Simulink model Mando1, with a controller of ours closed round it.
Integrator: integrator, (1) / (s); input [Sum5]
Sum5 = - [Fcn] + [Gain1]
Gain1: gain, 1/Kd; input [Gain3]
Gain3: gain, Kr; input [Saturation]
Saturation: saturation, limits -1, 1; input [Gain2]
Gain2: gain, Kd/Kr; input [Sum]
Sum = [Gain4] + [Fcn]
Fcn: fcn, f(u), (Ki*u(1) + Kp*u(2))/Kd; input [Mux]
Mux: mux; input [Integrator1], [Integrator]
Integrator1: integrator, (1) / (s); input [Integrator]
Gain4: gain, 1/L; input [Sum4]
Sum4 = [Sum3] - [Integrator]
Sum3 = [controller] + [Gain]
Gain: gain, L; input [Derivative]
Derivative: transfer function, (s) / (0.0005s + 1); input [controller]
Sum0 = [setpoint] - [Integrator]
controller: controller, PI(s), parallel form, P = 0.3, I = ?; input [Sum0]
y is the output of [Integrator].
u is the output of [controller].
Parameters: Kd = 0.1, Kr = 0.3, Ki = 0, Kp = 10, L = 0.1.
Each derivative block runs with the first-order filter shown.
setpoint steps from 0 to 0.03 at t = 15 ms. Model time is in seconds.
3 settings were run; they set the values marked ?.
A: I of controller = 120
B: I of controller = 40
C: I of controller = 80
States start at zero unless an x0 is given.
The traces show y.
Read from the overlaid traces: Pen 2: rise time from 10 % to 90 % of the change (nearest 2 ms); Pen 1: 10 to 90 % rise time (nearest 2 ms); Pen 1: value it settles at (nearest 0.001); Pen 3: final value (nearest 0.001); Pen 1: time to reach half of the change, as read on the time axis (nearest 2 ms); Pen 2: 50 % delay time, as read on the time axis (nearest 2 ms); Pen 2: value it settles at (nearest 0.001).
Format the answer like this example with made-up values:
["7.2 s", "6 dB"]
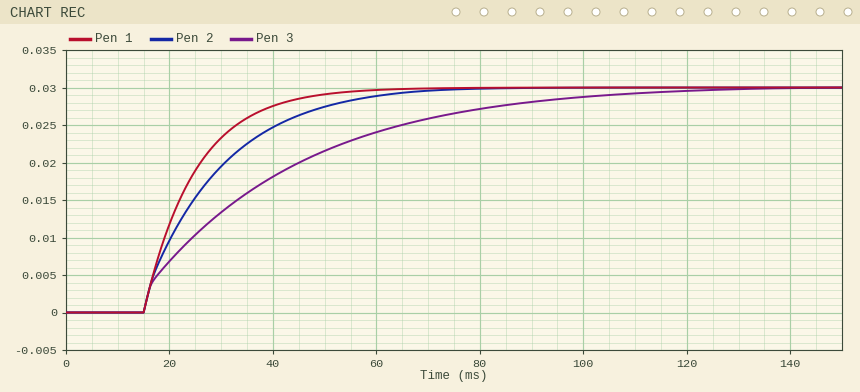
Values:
["32 ms", "22 ms", "0.030", "0.030", "22 ms", "24 ms", "0.030"]
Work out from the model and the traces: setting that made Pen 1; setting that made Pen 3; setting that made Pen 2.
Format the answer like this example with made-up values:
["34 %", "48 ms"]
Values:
["A", "B", "C"]
